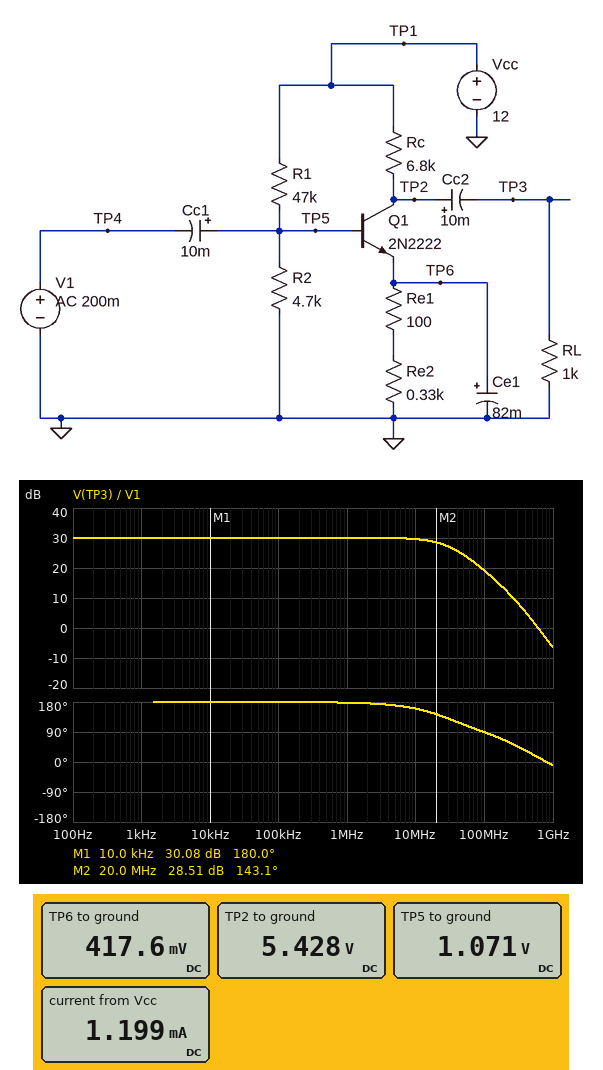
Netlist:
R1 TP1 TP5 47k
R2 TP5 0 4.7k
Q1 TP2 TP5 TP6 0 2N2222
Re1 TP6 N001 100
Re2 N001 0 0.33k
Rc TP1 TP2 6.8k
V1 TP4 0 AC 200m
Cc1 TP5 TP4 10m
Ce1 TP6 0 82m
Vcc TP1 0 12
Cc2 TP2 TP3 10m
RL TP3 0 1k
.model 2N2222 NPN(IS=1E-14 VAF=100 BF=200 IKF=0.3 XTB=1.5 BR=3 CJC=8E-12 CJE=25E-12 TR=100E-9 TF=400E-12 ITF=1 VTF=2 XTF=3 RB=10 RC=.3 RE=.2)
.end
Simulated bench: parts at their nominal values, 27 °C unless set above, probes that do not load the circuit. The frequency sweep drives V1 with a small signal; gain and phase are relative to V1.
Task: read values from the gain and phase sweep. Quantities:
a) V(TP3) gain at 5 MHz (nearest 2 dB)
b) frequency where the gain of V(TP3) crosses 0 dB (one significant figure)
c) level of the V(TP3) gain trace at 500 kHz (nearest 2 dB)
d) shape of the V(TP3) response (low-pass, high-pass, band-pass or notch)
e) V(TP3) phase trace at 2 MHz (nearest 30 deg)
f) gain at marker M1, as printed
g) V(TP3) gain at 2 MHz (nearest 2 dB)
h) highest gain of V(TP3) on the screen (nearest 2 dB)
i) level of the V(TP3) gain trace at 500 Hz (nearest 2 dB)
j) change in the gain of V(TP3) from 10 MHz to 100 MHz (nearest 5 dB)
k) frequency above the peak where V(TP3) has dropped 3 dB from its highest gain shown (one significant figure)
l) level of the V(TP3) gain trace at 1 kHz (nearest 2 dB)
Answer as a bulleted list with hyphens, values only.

- 30 dB
- 600 MHz
- 30 dB
- low-pass
- 180 deg
- 30.08 dB
- 30 dB
- 30 dB
- 30 dB
- -10 dB
- 30 MHz
- 30 dB
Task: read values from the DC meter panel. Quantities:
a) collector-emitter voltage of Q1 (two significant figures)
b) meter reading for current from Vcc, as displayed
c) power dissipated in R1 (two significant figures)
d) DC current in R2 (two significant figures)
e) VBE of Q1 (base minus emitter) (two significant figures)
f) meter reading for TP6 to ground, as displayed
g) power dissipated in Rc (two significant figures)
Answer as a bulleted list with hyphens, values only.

- 5.0 V
- 1.199 mA
- 2.5 mW
- 230 µA
- 650 mV
- 417.6 mV
- 6.4 mW
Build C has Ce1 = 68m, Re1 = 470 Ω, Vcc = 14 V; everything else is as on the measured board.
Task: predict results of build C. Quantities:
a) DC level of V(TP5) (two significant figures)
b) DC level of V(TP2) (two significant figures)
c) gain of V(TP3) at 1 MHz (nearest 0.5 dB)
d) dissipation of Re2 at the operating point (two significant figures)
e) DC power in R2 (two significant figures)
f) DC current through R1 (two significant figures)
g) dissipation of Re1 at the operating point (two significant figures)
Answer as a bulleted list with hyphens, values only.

- 1.3 V
- 8.8 V
- 28.0 dB
- 190 µW
- 340 µW
- 270 µA
- 270 µW
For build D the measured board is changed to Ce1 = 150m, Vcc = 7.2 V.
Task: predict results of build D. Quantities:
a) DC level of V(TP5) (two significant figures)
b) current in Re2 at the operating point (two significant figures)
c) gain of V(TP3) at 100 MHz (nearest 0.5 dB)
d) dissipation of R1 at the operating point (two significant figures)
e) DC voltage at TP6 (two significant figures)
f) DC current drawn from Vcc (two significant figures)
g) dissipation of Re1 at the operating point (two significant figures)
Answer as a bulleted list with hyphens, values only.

- 650 mV
- 120 µA
- 5.0 dB
- 910 µW
- 53 mV
- 260 µA
- 1.5 µW
